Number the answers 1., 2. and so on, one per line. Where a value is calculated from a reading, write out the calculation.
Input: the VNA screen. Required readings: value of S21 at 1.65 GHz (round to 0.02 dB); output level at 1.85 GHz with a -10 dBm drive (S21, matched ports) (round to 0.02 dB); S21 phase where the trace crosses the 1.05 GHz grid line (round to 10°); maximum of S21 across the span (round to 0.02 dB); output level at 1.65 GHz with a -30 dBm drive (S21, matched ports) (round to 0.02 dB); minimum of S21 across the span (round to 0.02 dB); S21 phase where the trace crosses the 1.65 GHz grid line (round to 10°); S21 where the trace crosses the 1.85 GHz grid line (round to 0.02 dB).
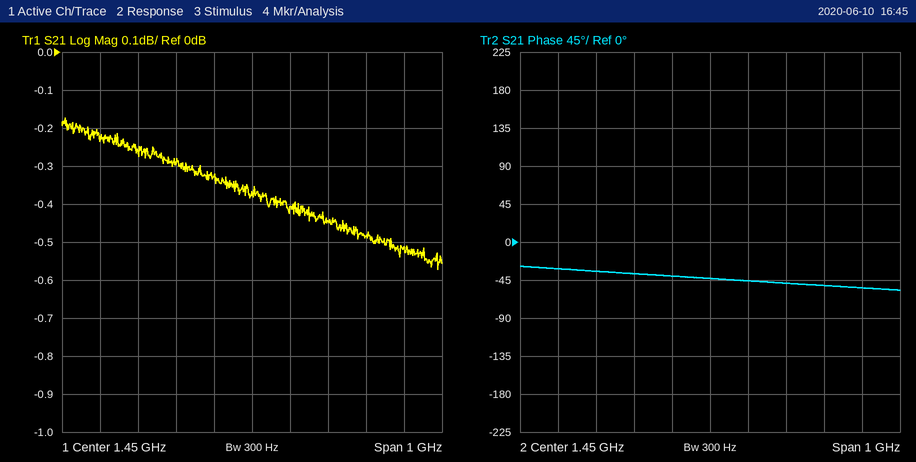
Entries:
1. -0.44 dB
2. -10 dBm + (-0.52 dB) = -10.52 dBm
3. -30°
4. -0.18 dB
5. -30 dBm + (-0.44 dB) = -30.44 dBm
6. -0.58 dB
7. -50°
8. -0.52 dB
